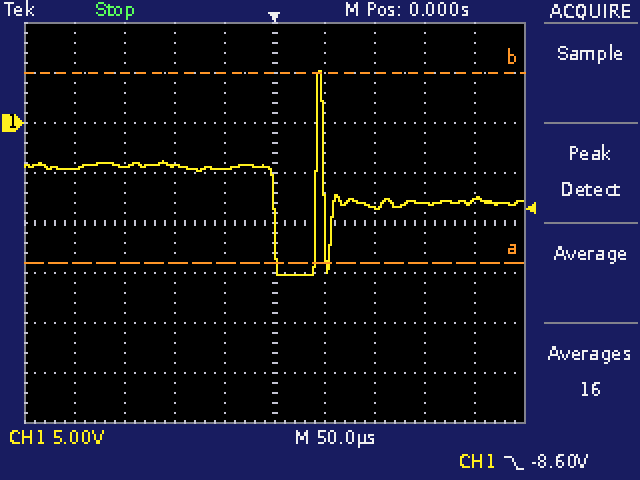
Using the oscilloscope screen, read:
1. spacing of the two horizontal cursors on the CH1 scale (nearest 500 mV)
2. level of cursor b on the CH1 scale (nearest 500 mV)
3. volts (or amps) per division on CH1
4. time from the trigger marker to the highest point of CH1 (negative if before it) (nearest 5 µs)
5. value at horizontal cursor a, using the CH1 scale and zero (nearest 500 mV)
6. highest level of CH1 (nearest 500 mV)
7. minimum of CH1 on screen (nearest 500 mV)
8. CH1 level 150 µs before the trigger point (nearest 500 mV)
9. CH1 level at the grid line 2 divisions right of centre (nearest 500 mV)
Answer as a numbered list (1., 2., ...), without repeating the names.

1. 19.0 V
2. 5.0 V
3. 5 V
4. +45 µs
5. -14.0 V
6. 5.0 V
7. -15.0 V
8. -4.5 V
9. -8.5 V
